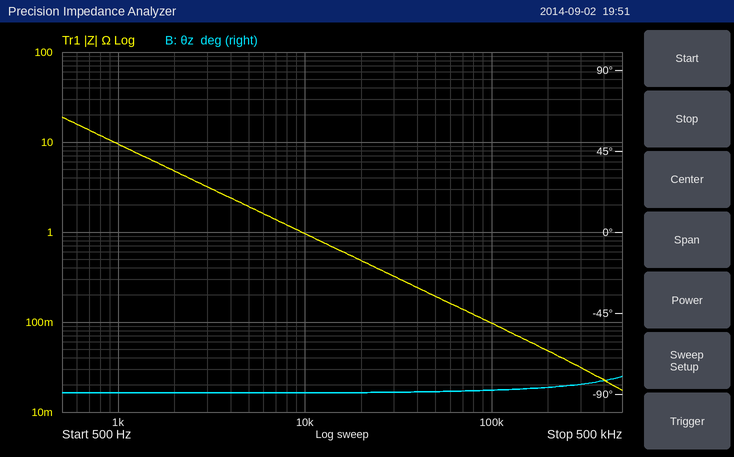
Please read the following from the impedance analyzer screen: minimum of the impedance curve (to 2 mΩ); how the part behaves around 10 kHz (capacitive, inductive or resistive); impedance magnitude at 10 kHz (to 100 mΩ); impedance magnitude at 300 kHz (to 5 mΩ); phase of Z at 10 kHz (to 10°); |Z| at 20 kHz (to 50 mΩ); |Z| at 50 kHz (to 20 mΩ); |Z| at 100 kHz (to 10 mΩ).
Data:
18 mΩ
capacitive
1.0 Ω
30 mΩ
-90°
500 mΩ
200 mΩ
100 mΩ
